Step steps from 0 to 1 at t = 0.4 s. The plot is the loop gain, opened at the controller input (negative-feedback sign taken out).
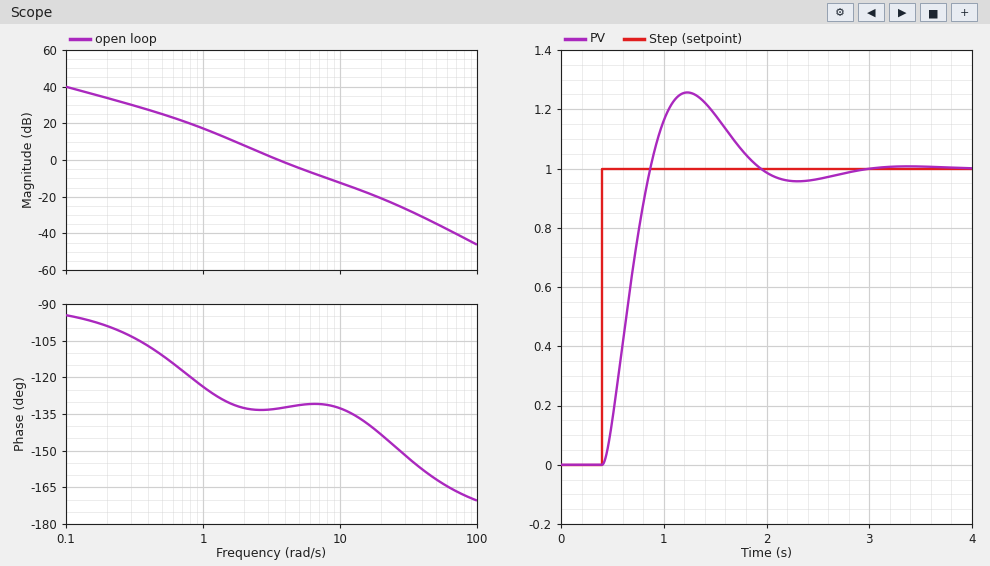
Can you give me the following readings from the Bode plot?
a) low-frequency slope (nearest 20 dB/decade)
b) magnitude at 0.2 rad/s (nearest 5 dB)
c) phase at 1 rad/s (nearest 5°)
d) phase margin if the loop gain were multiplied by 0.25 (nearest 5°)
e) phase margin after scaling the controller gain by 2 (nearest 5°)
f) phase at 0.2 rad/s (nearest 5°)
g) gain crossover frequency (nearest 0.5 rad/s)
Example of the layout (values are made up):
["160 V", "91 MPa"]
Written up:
["-20 dB/decade", "35 dB", "-125°", "50°", "50°", "-100°", "3.5 rad/s"]
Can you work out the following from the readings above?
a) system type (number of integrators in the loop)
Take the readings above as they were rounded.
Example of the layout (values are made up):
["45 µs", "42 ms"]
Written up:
["1"]
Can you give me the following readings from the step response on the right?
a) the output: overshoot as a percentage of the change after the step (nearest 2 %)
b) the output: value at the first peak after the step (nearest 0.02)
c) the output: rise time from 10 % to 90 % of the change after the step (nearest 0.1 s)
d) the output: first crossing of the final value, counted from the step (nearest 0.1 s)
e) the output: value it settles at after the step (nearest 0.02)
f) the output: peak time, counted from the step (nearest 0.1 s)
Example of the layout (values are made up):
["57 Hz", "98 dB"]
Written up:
["26 %", "1.26", "0.3 s", "0.5 s", "1.00", "0.8 s"]
